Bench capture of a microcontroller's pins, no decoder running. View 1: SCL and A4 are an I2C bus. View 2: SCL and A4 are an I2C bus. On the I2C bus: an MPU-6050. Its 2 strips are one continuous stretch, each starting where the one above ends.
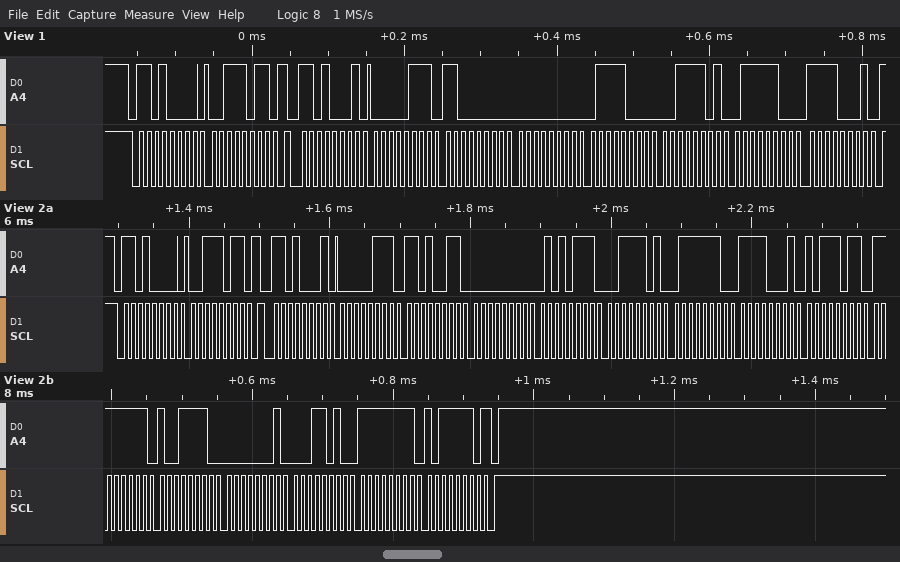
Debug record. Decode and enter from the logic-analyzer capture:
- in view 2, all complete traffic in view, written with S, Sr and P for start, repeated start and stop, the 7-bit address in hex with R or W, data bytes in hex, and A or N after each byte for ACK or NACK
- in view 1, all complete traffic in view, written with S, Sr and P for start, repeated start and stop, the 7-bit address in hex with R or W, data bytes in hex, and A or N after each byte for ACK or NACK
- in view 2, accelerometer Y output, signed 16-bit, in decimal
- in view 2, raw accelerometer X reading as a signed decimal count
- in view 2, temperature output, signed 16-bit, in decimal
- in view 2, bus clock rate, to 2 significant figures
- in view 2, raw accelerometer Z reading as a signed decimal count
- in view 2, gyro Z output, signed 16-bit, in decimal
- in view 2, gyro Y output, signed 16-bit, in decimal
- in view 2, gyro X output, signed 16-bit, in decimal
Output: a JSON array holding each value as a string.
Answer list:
["S 68W A 3B A Sr 68R A 07 A D3 A 00 A 57 A 3D A 7E A F1 A BB A FF A 9E A 01 A 1A A FF A BE N P", "S 68W A 3B A Sr 68R A 07 A C0 A 00 A 78 A 3D A 7C A F1 A", "87", "2003", "-3653", "100 kHz", "15742", "-66", "282", "-98"]
